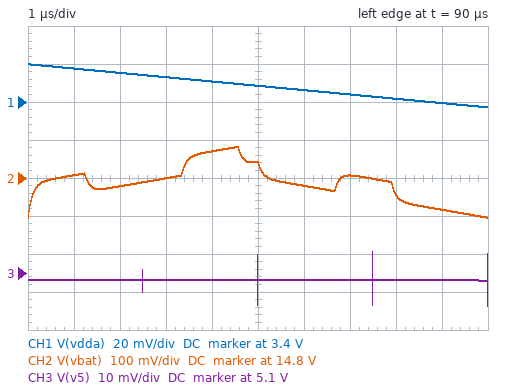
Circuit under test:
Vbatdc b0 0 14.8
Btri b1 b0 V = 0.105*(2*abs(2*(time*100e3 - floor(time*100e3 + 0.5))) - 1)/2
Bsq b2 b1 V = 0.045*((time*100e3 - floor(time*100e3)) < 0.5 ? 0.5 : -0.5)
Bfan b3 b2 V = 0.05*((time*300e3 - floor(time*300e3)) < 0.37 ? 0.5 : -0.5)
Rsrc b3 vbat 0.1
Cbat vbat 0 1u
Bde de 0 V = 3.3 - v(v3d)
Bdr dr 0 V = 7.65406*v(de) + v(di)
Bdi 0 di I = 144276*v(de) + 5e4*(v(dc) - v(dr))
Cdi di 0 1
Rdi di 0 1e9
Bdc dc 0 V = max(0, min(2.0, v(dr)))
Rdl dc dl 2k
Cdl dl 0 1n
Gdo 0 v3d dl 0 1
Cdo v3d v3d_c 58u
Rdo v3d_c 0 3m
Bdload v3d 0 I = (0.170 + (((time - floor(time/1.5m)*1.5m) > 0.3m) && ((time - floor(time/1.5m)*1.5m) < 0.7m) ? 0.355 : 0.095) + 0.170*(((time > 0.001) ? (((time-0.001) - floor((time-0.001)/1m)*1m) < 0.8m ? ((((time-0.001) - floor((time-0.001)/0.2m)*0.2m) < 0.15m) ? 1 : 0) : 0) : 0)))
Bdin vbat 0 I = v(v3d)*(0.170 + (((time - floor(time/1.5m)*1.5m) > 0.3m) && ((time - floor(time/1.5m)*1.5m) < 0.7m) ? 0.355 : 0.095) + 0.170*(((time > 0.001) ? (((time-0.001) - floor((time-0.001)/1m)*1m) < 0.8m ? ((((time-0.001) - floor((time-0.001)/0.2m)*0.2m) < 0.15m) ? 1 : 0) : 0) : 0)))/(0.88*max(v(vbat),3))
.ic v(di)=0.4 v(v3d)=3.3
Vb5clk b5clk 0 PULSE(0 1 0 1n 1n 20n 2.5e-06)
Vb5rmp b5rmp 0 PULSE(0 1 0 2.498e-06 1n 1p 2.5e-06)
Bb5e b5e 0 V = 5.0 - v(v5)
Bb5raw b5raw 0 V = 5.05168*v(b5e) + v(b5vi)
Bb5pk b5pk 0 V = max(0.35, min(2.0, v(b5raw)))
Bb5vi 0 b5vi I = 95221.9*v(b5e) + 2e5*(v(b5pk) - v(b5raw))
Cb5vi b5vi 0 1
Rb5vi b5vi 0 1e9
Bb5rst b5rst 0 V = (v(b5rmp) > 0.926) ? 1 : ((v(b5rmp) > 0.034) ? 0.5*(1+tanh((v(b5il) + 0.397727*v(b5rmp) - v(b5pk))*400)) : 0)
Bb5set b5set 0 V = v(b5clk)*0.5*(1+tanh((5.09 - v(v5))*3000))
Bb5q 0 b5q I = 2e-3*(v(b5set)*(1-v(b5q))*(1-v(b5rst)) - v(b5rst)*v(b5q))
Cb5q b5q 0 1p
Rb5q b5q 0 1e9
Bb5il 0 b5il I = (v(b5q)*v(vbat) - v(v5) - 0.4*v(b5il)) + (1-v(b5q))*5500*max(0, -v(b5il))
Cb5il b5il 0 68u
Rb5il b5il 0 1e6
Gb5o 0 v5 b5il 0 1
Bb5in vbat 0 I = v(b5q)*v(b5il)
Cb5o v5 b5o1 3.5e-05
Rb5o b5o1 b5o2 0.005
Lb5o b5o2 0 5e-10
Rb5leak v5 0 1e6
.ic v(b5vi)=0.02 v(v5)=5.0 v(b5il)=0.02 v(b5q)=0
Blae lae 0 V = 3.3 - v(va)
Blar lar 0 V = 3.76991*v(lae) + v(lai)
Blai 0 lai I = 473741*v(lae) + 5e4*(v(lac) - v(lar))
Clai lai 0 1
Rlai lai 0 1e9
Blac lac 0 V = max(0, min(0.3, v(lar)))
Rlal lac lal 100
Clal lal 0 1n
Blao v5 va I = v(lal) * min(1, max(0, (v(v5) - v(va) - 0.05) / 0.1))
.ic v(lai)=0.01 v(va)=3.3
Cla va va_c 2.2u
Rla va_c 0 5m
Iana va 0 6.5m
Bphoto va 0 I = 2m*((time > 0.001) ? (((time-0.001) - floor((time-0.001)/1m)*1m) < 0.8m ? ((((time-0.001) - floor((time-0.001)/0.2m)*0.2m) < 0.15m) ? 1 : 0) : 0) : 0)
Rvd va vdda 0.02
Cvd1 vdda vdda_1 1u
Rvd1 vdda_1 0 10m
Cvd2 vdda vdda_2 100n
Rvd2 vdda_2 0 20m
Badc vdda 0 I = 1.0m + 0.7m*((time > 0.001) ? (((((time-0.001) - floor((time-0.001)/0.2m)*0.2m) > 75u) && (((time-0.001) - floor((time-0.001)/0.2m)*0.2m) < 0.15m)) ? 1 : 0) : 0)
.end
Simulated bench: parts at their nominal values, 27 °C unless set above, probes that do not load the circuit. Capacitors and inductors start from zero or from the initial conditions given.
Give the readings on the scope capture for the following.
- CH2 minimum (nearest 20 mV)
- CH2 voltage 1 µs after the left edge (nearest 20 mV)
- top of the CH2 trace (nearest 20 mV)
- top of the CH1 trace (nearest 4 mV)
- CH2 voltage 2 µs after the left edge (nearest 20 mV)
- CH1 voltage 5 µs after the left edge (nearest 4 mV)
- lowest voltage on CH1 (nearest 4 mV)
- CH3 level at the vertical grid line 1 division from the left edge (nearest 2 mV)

14.70 V
14.80 V
14.88 V
3.420 V
14.78 V
3.408 V
3.396 V
5.098 V
